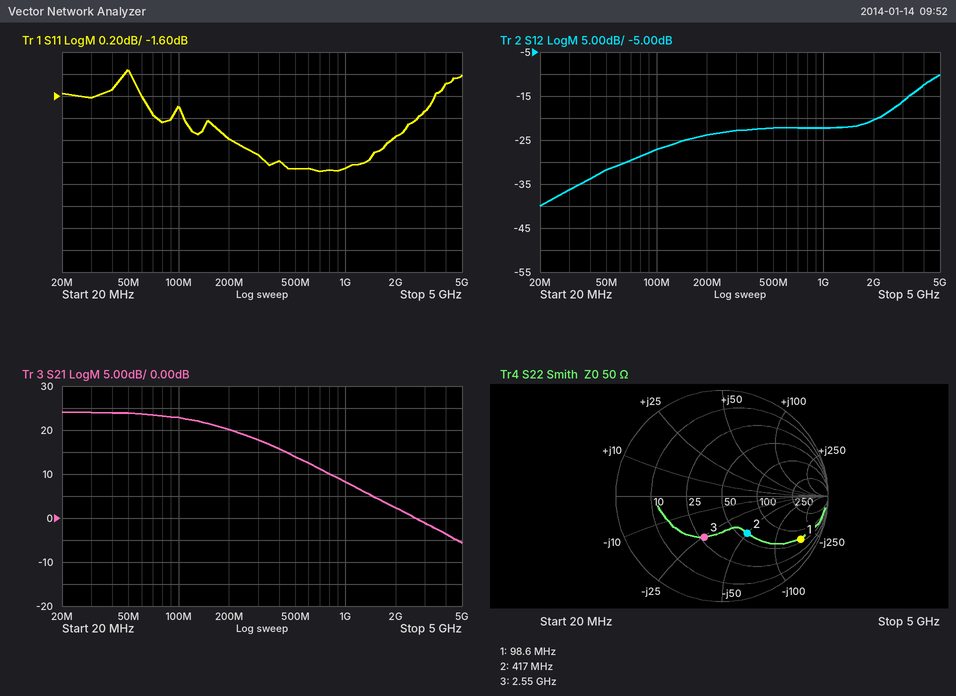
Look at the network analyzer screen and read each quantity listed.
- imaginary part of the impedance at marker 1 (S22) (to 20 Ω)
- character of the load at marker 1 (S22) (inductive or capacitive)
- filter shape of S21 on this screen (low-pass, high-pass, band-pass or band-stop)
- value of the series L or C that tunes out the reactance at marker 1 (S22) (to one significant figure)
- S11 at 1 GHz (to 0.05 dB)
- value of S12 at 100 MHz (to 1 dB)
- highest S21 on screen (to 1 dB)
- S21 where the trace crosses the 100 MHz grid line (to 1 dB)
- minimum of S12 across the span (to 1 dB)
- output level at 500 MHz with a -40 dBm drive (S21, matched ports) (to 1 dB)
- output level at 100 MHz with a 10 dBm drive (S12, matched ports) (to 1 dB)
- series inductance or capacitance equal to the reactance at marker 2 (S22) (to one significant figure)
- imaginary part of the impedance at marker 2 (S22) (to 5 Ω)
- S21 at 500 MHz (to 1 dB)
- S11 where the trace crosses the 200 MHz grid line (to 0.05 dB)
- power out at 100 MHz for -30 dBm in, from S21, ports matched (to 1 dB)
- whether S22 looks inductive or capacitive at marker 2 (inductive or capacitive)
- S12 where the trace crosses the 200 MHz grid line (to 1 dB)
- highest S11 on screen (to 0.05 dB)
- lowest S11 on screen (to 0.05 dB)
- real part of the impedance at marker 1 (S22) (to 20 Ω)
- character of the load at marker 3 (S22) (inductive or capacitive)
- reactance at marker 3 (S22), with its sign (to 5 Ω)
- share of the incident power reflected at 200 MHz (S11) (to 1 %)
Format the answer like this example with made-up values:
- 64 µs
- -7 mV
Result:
- -180 Ω
- capacitive
- low-pass
- 300 nH
- -2.25 dB
- -27 dB
- 24 dB
- 23 dB
- -40 dB
- -26 dBm
- -17 dBm
- 8 pF
- -50 Ω
- 14 dB
- -2.00 dB
- -7 dBm
- capacitive
- -24 dB
- -1.35 dB
- -2.30 dB
- 60 Ω
- capacitive
- -25 Ω
- 63 %
